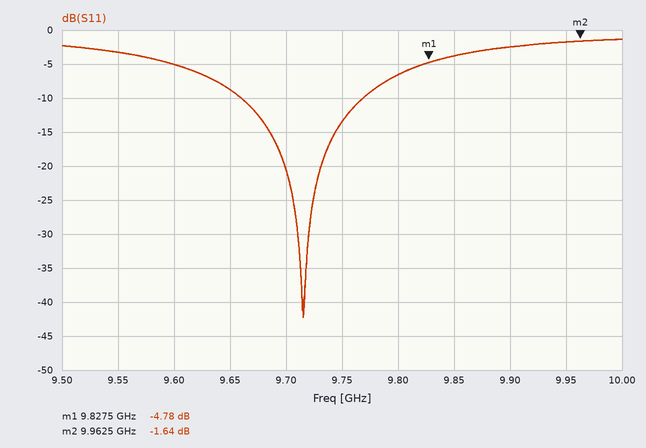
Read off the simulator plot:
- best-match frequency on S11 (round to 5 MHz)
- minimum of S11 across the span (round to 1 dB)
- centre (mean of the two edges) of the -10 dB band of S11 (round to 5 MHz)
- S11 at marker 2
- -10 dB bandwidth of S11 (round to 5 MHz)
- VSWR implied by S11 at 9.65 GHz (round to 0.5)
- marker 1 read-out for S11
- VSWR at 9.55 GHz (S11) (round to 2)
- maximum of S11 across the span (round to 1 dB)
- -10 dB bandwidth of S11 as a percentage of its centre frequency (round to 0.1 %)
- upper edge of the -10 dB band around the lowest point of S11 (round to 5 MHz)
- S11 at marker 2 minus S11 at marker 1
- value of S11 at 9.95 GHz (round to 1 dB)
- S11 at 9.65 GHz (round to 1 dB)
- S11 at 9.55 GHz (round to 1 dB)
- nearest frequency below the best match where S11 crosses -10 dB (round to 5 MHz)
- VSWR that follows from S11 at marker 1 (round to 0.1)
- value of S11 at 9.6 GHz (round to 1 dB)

9.715 GHz
-42 dB
9.715 GHz
-1.64 dB
110 MHz
2.0
-4.78 dB
6
-1 dB
1.1 %
9.770 GHz
3.14 dB
-2 dB
-9 dB
-3 dB
9.660 GHz
3.7
-5 dB
